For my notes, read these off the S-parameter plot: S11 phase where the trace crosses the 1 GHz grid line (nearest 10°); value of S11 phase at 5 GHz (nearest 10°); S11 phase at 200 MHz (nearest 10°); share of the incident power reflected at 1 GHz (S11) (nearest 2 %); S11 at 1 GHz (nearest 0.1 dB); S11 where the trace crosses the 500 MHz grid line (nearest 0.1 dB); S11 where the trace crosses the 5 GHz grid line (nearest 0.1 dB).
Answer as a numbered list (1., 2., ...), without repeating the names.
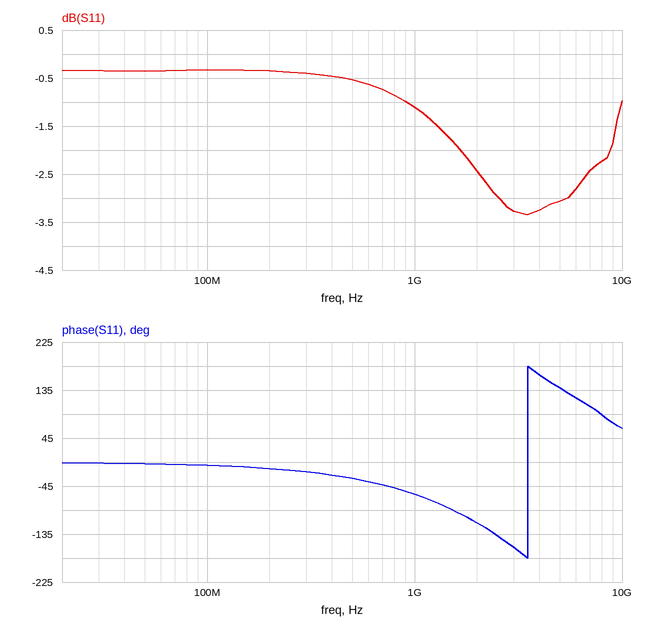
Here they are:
1. -60°
2. 140°
3. -10°
4. 78 %
5. -1.1 dB
6. -0.5 dB
7. -3.1 dB
